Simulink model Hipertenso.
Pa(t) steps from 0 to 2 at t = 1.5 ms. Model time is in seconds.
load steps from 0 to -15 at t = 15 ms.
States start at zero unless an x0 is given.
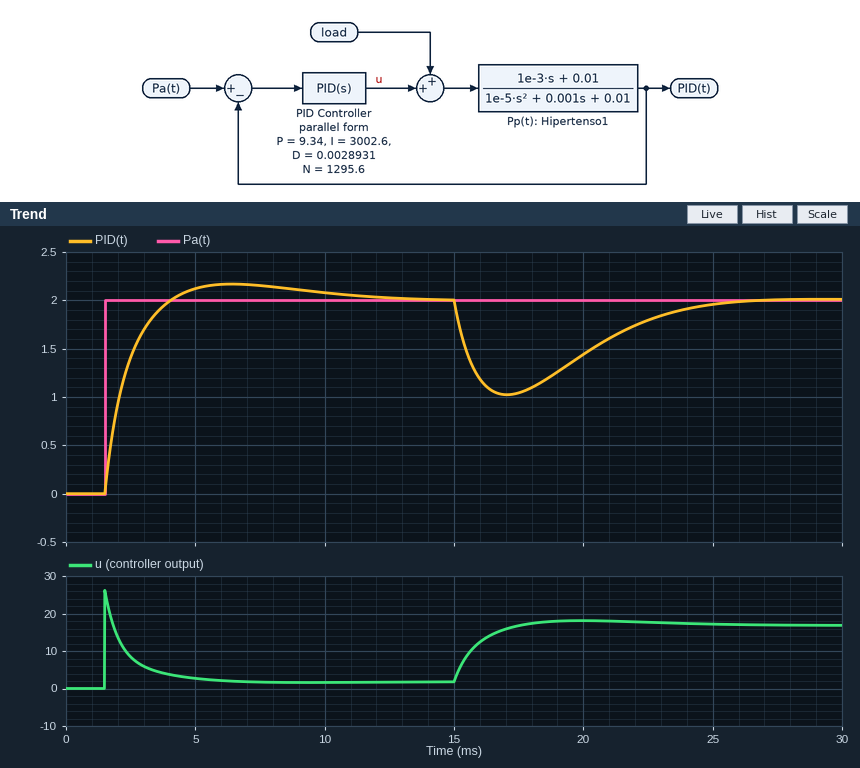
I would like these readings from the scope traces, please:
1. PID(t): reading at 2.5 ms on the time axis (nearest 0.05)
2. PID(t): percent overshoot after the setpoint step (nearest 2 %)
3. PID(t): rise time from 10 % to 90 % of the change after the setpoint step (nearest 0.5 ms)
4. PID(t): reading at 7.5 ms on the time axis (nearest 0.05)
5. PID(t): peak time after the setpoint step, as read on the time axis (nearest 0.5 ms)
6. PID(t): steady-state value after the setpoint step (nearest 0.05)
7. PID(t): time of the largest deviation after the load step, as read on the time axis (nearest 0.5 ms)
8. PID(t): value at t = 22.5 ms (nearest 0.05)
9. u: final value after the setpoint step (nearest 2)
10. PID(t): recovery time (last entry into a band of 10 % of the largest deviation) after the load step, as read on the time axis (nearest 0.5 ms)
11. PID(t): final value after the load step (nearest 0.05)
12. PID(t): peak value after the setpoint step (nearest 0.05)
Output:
1.40
8 %
1.5 ms
2.15
6.5 ms
2.00
17.0 ms
1.80
2
24.0 ms
2.00
2.15
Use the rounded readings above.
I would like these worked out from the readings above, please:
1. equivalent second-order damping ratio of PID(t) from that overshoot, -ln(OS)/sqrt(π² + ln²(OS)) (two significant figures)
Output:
0.63
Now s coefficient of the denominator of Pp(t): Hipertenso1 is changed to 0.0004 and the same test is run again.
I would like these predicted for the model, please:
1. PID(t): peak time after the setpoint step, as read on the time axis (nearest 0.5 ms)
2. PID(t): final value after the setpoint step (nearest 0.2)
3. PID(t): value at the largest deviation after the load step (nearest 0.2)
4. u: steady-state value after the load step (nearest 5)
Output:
6.0 ms
2.0
1.0
15
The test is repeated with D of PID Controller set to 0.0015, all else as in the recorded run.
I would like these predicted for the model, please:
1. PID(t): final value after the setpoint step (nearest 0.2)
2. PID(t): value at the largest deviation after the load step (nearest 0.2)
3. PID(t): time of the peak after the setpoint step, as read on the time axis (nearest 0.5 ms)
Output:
2.0
1.0
6.0 ms
